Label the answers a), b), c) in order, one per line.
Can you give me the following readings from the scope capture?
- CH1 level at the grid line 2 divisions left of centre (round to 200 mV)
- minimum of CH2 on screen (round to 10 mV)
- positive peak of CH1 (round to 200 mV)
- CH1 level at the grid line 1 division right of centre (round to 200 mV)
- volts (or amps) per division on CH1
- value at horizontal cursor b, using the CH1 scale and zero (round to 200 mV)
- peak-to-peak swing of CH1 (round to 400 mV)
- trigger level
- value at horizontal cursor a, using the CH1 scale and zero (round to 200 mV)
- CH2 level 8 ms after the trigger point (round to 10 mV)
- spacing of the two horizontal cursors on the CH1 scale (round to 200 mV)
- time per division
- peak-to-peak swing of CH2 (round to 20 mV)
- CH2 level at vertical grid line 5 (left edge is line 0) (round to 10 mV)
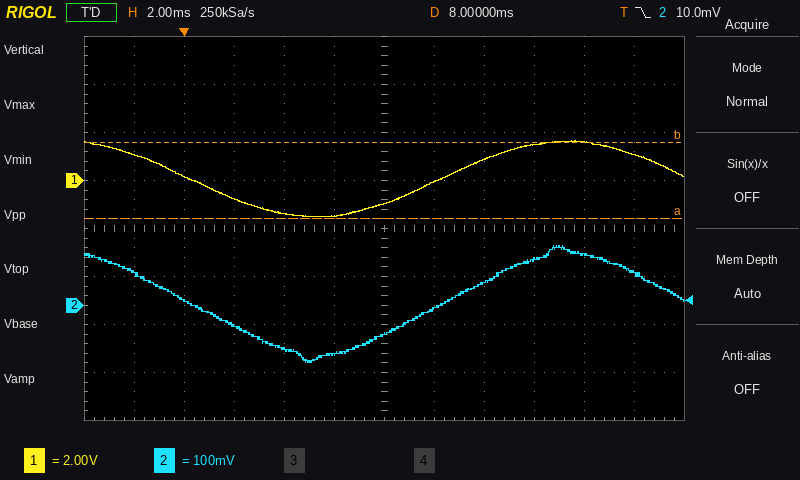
a) -1.4 V
b) -120 mV
c) 1.6 V
d) 0.0 V
e) 2 V
f) 1.6 V
g) 3.2 V
h) 10.0 mV
i) -1.6 V
j) -60 mV
k) 3.2 V
l) 2 ms
m) 240 mV
n) -100 mV
